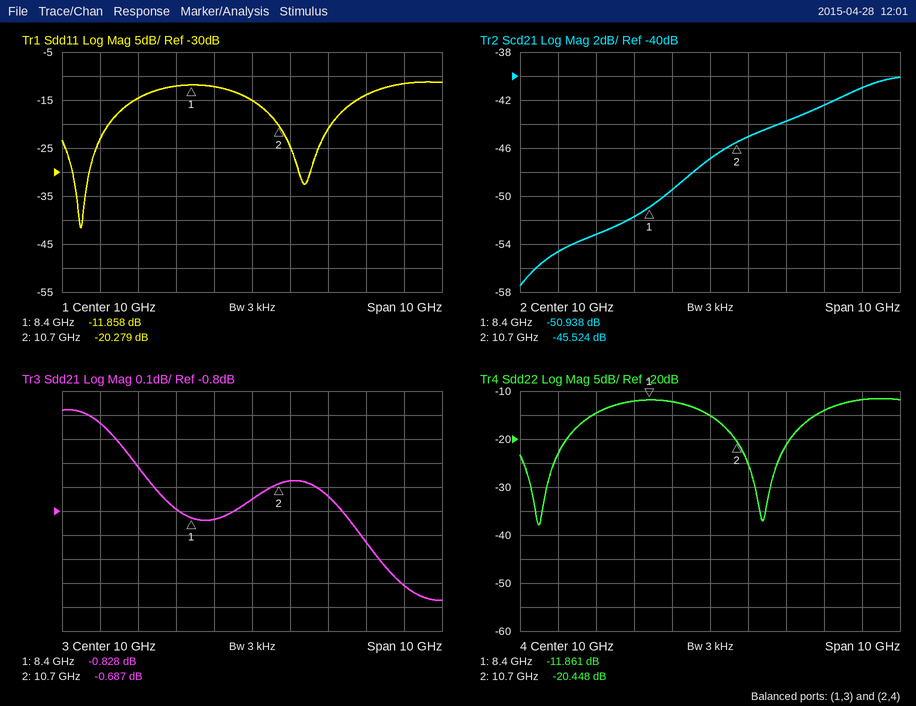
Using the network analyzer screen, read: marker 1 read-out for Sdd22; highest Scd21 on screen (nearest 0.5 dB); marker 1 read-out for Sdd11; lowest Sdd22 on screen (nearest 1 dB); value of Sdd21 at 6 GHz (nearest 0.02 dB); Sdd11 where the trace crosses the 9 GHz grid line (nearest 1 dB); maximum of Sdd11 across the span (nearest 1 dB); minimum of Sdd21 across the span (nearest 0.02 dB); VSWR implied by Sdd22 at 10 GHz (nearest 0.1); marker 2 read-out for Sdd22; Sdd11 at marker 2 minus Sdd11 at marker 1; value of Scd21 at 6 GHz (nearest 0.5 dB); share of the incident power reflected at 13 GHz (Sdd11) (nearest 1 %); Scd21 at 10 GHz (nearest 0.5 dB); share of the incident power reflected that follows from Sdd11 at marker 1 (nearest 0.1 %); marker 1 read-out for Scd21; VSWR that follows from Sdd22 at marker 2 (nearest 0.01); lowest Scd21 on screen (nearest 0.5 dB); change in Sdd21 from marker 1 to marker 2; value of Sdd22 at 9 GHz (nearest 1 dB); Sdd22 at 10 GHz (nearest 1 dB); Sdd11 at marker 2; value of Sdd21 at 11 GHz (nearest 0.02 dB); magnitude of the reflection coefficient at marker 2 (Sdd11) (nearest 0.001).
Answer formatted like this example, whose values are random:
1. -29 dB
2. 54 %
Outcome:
1. -11.861 dB
2. -40.0 dB
3. -11.858 dB
4. -38 dB
5. -0.44 dB
6. -12 dB
7. -11 dB
8. -1.18 dB
9. 1.4
10. -20.448 dB
11. -8.421 dB
12. -54.5 dB
13. 4 %
14. -47.0 dB
15. 6.5 %
16. -50.938 dB
17. 1.21
18. -57.5 dB
19. 0.141 dB
20. -12 dB
21. -15 dB
22. -20.279 dB
23. -0.68 dB
24. 0.097
